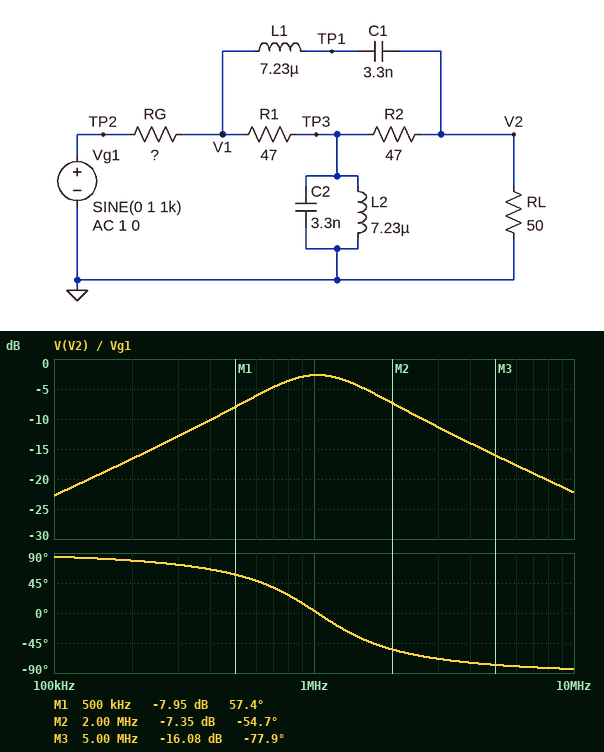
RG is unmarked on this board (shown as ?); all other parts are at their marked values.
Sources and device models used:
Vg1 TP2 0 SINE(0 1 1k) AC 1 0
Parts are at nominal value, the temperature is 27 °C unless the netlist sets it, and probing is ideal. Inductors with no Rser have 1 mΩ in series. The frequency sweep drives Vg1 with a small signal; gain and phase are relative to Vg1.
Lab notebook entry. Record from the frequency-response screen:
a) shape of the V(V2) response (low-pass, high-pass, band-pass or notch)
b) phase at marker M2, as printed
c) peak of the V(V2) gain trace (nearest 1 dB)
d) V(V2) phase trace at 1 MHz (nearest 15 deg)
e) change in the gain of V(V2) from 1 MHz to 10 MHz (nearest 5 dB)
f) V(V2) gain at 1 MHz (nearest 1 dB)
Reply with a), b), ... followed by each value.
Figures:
a) band-pass
b) -54.7 deg
c) -3 dB
d) 0 deg
e) -20 dB
f) -3 dB
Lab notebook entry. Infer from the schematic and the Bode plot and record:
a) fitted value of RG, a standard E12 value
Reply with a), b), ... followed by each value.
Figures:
a) 18 Ω
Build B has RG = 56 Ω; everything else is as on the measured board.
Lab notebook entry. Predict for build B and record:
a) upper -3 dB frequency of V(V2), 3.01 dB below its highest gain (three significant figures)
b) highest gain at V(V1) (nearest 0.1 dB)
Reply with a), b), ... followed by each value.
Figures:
a) 1.66 MHz
b) -6.5 dB
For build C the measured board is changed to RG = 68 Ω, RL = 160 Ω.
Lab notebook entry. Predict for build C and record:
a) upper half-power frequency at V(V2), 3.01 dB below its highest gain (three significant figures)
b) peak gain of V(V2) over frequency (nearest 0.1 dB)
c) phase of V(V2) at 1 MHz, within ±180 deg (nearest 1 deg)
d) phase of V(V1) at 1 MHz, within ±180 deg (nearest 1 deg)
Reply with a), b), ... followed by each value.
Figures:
a) 1.53 MHz
b) -3.1 dB
c) 4 deg
d) 3 deg
